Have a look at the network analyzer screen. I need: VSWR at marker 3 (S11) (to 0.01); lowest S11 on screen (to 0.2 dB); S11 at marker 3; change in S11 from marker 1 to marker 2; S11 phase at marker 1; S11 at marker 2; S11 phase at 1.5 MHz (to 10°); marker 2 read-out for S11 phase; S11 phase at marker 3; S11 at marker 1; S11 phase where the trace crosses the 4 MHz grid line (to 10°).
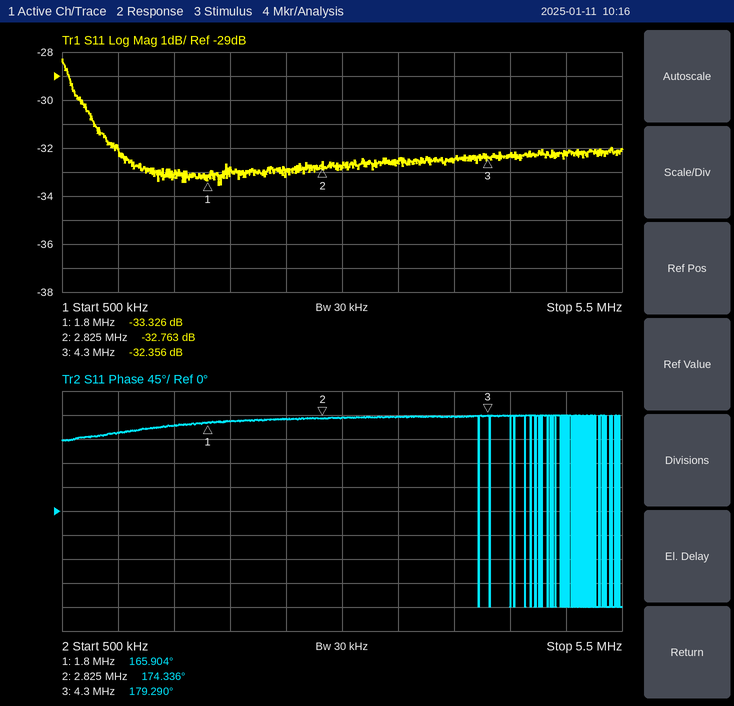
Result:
1.05
-33.6 dB
-32.356 dB
0.563 dB
165.904°
-32.763 dB
160°
174.336°
179.290°
-33.326 dB
180°
